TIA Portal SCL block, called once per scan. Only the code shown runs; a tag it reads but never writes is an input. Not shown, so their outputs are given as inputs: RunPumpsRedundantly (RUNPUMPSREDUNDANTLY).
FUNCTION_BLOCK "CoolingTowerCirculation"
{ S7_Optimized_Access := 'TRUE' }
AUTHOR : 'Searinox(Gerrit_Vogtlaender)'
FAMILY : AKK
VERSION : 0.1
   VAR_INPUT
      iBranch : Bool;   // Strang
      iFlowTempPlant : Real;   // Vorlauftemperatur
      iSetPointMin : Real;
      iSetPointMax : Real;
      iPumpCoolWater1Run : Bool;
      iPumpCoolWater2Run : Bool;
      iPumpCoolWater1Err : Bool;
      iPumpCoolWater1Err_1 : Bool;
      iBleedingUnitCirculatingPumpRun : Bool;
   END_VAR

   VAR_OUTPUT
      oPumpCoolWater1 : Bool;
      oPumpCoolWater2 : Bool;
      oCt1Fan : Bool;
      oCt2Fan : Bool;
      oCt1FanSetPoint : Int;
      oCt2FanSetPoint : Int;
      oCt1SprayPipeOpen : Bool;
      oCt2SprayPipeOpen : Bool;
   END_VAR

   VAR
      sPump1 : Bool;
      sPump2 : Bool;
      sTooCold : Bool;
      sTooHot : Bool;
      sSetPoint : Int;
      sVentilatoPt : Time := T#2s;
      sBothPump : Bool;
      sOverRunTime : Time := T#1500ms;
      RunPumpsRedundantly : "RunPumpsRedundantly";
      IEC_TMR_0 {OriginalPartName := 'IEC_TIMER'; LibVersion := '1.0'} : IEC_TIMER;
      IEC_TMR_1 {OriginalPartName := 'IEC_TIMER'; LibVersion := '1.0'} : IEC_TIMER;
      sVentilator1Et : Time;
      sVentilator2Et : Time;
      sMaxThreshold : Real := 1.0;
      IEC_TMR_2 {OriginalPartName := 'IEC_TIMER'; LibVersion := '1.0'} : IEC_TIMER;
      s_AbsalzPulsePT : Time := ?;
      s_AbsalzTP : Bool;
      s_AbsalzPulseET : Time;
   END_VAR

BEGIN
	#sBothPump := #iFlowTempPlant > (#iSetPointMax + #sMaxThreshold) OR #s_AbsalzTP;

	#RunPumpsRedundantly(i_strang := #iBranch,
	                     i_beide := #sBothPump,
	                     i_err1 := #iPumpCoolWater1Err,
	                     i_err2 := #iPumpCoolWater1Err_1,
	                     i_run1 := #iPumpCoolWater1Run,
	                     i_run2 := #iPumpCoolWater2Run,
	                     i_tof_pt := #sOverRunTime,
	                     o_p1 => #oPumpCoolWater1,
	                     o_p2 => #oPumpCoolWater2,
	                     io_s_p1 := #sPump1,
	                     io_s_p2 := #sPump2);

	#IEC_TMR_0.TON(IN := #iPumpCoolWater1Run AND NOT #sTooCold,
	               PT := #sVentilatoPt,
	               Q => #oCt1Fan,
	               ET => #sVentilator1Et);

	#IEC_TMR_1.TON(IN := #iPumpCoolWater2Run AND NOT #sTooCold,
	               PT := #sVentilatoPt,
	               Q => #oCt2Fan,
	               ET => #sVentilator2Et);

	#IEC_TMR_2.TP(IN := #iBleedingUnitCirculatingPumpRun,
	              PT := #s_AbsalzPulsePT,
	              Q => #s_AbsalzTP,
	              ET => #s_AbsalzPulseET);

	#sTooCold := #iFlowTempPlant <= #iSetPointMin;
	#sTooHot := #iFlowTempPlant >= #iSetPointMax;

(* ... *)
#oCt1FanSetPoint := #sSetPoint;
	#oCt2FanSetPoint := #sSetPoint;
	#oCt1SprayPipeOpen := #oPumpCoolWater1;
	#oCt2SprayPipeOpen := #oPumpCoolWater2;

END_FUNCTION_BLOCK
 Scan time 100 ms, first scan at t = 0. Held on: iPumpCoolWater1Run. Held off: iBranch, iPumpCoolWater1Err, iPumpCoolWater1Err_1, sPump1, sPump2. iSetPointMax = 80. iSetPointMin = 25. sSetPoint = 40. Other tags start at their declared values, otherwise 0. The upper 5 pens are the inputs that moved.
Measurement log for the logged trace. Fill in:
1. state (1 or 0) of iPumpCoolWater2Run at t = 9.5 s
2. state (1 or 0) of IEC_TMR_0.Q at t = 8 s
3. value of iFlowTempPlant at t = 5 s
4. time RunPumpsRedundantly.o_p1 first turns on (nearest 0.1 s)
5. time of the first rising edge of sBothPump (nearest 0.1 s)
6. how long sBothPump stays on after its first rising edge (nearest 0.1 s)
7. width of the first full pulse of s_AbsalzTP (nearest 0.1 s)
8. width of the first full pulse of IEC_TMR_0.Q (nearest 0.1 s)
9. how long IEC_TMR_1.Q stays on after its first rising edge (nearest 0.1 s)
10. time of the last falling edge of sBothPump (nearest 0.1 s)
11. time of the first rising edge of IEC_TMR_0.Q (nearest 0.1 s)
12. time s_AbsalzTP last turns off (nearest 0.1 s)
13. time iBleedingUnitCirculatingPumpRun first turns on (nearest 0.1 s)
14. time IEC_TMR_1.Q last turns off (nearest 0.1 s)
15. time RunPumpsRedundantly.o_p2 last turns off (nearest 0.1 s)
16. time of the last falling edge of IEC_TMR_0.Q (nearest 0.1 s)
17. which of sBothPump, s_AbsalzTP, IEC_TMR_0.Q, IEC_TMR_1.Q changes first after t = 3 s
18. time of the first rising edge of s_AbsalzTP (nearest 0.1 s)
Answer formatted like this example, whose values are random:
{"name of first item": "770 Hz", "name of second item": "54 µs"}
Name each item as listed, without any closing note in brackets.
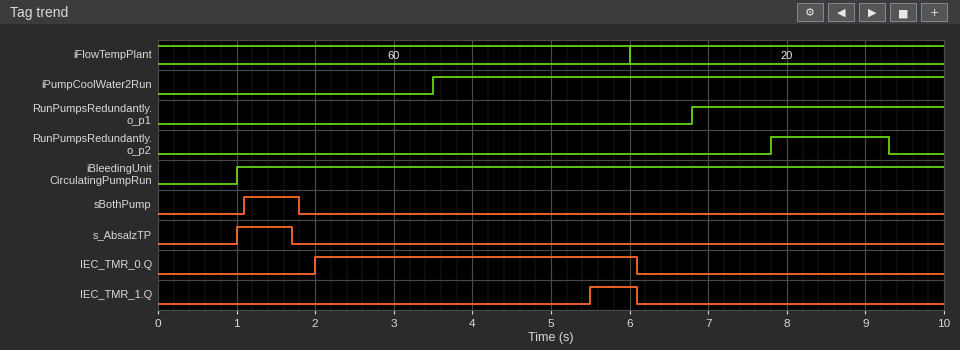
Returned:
{"state (1 or 0) of iPumpCoolWater2Run at t = 9.5 s": "1", "state (1 or 0) of IEC_TMR_0.Q at t = 8 s": "0", "value of iFlowTempPlant at t = 5 s": "60", "time RunPumpsRedundantly.o_p1 first turns on": "6.8 s", "time of the first rising edge of sBothPump": "1.1 s", "how long sBothPump stays on after its first rising edge": "0.7 s", "width of the first full pulse of s_AbsalzTP": "0.7 s", "width of the first full pulse of IEC_TMR_0.Q": "4.1 s", "how long IEC_TMR_1.Q stays on after its first rising edge": "0.6 s", "time of the last falling edge of sBothPump": "1.8 s", "time of the first rising edge of IEC_TMR_0.Q": "2.0 s", "time s_AbsalzTP last turns off": "1.7 s", "time iBleedingUnitCirculatingPumpRun first turns on": "1.0 s", "time IEC_TMR_1.Q last turns off": "6.1 s", "time RunPumpsRedundantly.o_p2 last turns off": "9.3 s", "time of the last falling edge of IEC_TMR_0.Q": "6.1 s", "which of sBothPump, s_AbsalzTP, IEC_TMR_0.Q, IEC_TMR_1.Q changes first after t = 3 s": "IEC_TMR_1.Q", "time of the first rising edge of s_AbsalzTP": "1.0 s"}
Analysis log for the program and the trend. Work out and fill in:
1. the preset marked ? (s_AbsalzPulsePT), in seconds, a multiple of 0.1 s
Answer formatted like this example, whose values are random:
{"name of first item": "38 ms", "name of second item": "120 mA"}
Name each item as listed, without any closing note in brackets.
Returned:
{"the preset marked ? (s_AbsalzPulsePT), in seconds, a multiple of 0.1 s": "0.7 s"}
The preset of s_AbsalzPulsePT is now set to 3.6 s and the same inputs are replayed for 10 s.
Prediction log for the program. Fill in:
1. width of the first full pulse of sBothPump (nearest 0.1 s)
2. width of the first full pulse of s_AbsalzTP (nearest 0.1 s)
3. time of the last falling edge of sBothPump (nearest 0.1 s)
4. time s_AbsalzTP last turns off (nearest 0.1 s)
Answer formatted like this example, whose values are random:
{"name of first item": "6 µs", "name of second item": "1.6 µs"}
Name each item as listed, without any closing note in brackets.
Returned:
{"width of the first full pulse of sBothPump": "3.6 s", "width of the first full pulse of s_AbsalzTP": "3.6 s", "time of the last falling edge of sBothPump": "4.7 s", "time s_AbsalzTP last turns off": "4.6 s"}
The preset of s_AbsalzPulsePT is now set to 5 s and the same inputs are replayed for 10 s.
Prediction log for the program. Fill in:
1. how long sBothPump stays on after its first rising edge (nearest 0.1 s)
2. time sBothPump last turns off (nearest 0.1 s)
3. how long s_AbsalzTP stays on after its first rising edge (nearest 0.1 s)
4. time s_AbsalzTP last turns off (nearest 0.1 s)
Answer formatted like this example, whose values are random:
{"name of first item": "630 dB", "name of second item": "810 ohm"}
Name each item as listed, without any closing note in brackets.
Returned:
{"how long sBothPump stays on after its first rising edge": "5.0 s", "time sBothPump last turns off": "6.1 s", "how long s_AbsalzTP stays on after its first rising edge": "5.0 s", "time s_AbsalzTP last turns off": "6.0 s"}
